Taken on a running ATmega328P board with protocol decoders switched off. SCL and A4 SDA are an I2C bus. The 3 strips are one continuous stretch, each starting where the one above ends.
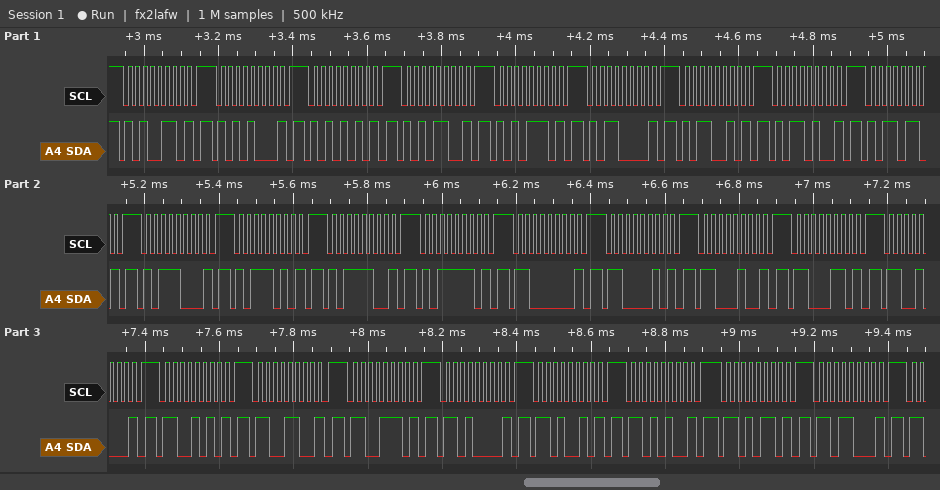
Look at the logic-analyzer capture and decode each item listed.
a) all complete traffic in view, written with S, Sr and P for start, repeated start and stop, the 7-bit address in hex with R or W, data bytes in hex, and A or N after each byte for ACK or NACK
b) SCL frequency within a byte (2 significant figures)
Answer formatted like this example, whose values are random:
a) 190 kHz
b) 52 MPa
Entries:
a) S 53W N P S 54W N P S 55W N P S 56W N P S 57W N P S 58W N P S 59W N P S 5AW N P S 5BW N P S 5CW N P S 5DW N P S 5EW N P S 5FW N P S 60W N P S 61W N P S 62W N P S 63W N P S 64W N P S 65W N P S 66W N P S 67W N P S 68W N P S 69W N P S 6AW N P S 6BW N P S 6CW N P
b) 50 kHz
